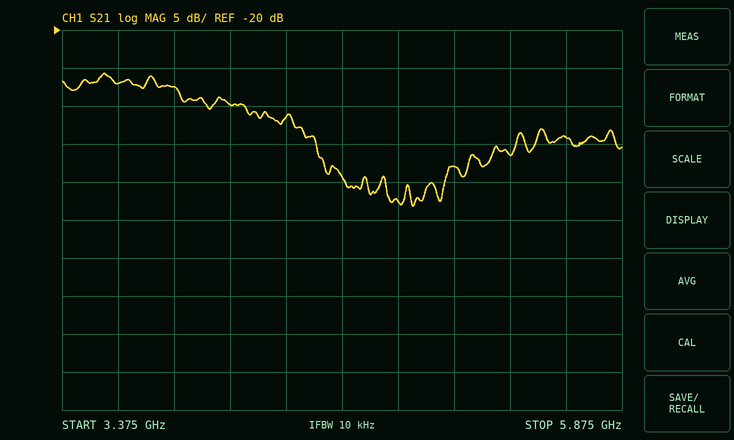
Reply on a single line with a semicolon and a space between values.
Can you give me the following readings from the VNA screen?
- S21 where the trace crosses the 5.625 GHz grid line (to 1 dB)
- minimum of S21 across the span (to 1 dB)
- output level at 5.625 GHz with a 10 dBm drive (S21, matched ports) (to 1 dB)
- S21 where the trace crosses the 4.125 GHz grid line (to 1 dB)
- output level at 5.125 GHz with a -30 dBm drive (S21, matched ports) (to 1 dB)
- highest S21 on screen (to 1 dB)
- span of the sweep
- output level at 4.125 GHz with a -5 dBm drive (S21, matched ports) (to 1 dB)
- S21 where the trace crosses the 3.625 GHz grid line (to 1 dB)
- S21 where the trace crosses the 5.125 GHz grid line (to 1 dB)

-34 dB; -43 dB; -24 dBm; -30 dB; -68 dBm; -26 dB; 2.5 GHz; -35 dBm; -27 dB; -38 dB
